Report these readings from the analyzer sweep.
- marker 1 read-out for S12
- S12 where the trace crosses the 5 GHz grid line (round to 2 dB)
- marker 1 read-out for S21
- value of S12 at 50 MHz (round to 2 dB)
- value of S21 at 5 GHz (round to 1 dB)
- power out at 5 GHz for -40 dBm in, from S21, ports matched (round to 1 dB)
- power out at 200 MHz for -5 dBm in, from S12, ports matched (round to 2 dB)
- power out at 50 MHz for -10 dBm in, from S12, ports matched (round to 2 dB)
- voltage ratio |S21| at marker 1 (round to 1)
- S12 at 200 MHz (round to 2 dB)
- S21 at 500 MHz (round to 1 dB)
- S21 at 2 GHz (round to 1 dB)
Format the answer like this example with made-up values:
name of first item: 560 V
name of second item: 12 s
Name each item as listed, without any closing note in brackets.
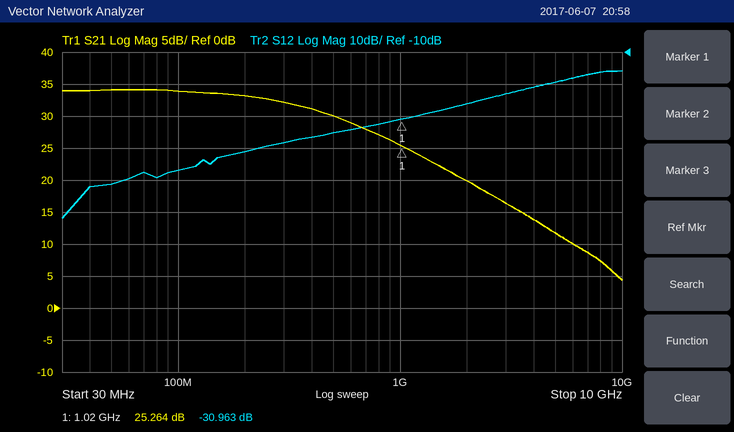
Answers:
marker 1 read-out for S12: -30.963 dB
S12 where the trace crosses the 5 GHz grid line: -20 dB
marker 1 read-out for S21: 25.264 dB
value of S12 at 50 MHz: -52 dB
value of S21 at 5 GHz: 12 dB
power out at 5 GHz for -40 dBm in, from S21, ports matched: -28 dBm
power out at 200 MHz for -5 dBm in, from S12, ports matched: -46 dBm
power out at 50 MHz for -10 dBm in, from S12, ports matched: -62 dBm
voltage ratio |S21| at marker 1: 18
S12 at 200 MHz: -42 dB
S21 at 500 MHz: 30 dB
S21 at 2 GHz: 20 dB
